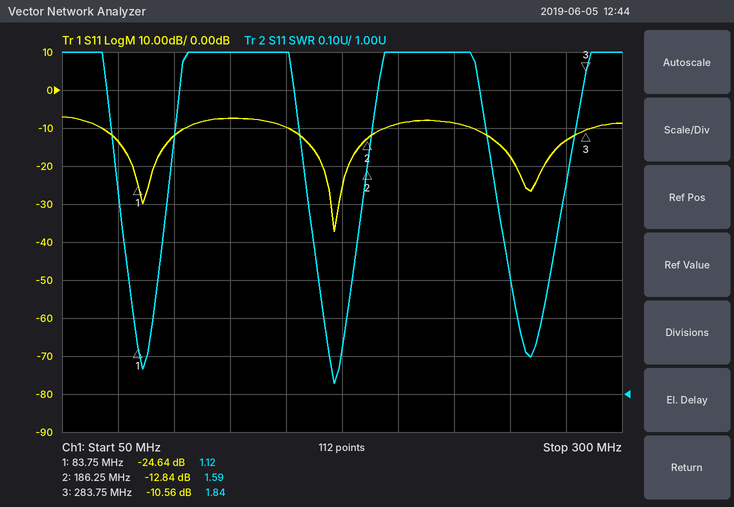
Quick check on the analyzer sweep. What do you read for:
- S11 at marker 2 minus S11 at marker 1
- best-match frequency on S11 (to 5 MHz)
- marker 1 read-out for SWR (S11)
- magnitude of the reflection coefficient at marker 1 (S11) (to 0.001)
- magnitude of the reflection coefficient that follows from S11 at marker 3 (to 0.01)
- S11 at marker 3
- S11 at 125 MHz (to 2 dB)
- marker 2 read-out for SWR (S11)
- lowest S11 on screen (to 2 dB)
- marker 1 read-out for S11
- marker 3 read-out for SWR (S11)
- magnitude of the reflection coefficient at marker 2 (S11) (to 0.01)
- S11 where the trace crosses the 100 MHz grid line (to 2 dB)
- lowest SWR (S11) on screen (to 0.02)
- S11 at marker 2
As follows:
11.80 dB
170 MHz
1.12
0.059
0.30
-10.56 dB
-8 dB
1.59
-38 dB
-24.64 dB
1.84
0.23
-12 dB
1.02
-12.84 dB
